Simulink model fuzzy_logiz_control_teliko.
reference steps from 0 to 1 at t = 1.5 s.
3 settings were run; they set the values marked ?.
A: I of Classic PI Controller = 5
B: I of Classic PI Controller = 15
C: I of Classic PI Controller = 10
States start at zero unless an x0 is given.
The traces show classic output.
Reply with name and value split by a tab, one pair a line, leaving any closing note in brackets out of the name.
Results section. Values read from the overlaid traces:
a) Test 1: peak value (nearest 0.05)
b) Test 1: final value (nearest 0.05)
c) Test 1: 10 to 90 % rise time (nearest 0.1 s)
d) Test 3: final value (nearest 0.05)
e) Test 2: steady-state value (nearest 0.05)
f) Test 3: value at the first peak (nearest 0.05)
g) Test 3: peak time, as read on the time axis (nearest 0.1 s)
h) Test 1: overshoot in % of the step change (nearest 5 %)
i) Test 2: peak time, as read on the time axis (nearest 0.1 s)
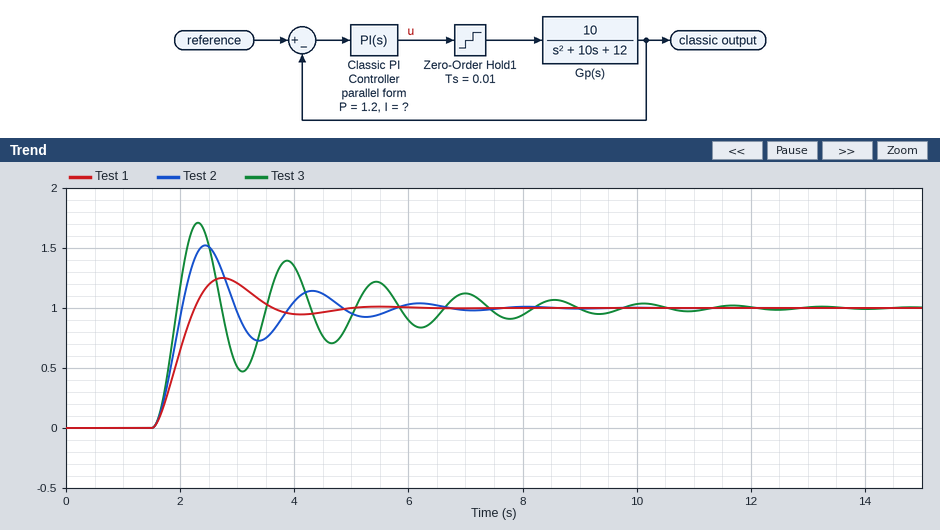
Test 1: peak value	1.25
Test 1: final value	1.00
Test 1: 10 to 90 % rise time	0.5 s
Test 3: final value	1.00
Test 2: steady-state value	1.00
Test 3: value at the first peak	1.70
Test 3: peak time, as read on the time axis	2.3 s
Test 1: overshoot in % of the step change	25 %
Test 2: peak time, as read on the time axis	2.4 s
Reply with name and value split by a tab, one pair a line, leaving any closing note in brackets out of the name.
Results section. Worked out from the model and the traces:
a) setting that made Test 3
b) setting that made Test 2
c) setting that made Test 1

setting that made Test 3	B
setting that made Test 2	C
setting that made Test 1	A
